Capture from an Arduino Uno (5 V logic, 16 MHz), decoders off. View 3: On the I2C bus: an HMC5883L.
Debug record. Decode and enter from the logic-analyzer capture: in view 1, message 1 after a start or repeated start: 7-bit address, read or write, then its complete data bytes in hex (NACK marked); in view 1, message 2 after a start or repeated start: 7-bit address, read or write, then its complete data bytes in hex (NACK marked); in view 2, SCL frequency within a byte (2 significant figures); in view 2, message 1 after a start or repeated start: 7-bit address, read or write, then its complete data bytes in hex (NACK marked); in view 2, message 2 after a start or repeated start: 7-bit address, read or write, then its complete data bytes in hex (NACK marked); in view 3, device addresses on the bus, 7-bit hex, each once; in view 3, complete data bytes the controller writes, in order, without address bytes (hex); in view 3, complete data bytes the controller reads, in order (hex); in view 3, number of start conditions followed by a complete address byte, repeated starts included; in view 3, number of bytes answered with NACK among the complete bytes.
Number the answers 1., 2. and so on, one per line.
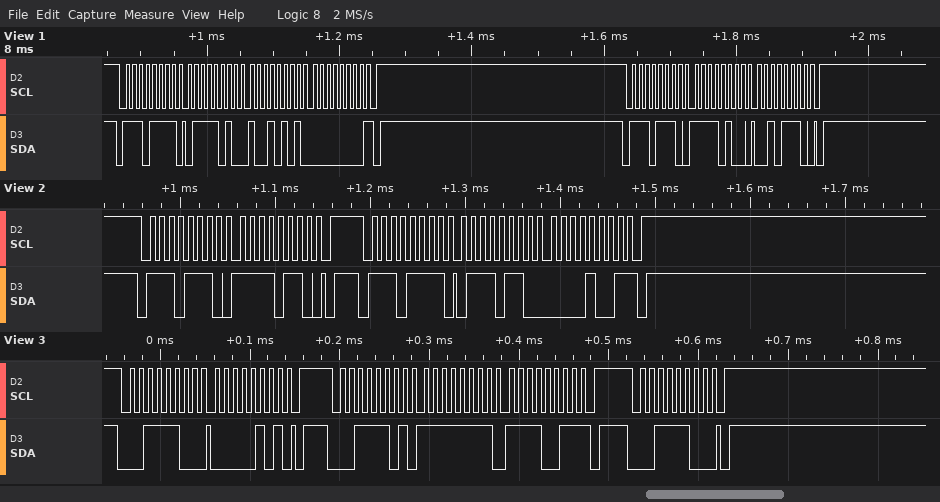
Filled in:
1. 0x77 read: 7A 95 00 NACK
2. 0x77 write: F4 2E
3. 100 kHz
4. 0x77 write: F6
5. 0x77 read: 76 09 NACK
6. 0x1E
7. 05
8. FF F3
9. 3
10. 1
